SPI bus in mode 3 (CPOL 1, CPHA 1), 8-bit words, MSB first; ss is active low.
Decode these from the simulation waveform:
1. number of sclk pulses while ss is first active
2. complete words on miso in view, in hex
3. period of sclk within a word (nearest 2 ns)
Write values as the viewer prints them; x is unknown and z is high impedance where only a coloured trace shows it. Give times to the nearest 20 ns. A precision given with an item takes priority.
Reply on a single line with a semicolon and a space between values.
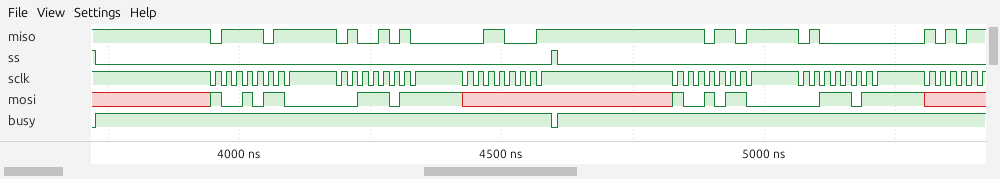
24; 7B, 4A, 31, ED, 40; 20 ns
